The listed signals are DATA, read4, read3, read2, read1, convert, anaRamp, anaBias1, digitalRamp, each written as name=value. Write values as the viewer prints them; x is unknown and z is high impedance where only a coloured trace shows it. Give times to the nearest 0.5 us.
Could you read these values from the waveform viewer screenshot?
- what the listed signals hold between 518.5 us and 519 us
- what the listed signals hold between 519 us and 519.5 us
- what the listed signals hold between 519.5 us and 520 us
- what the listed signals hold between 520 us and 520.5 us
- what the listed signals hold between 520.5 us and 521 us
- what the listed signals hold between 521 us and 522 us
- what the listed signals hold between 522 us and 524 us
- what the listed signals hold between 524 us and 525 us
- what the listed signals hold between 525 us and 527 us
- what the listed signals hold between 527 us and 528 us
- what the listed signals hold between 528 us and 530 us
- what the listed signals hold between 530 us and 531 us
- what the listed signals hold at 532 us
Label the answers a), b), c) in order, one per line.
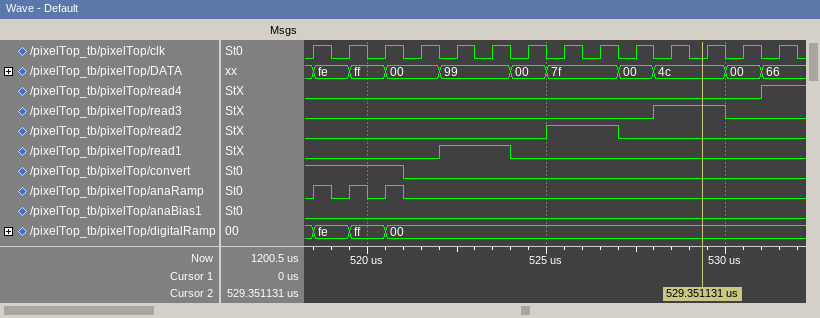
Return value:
a) DATA=fe, read4=0, read3=0, read2=0, read1=0, convert=1, anaRamp=1, anaBias1=0, digitalRamp=fe
b) DATA=fe, read4=0, read3=0, read2=0, read1=0, convert=1, anaRamp=0, anaBias1=0, digitalRamp=fe
c) DATA=ff, read4=0, read3=0, read2=0, read1=0, convert=1, anaRamp=1, anaBias1=0, digitalRamp=ff
d) DATA=ff, read4=0, read3=0, read2=0, read1=0, convert=1, anaRamp=0, anaBias1=0, digitalRamp=ff
e) DATA=00, read4=0, read3=0, read2=0, read1=0, convert=1, anaRamp=1, anaBias1=0, digitalRamp=00
f) DATA=00, read4=0, read3=0, read2=0, read1=0, convert=0, anaRamp=0, anaBias1=0, digitalRamp=00
g) DATA=99, read4=0, read3=0, read2=0, read1=1, convert=0, anaRamp=0, anaBias1=0, digitalRamp=00
h) DATA=00, read4=0, read3=0, read2=0, read1=0, convert=0, anaRamp=0, anaBias1=0, digitalRamp=00
i) DATA=7f, read4=0, read3=0, read2=1, read1=0, convert=0, anaRamp=0, anaBias1=0, digitalRamp=00
j) DATA=00, read4=0, read3=0, read2=0, read1=0, convert=0, anaRamp=0, anaBias1=0, digitalRamp=00
k) DATA=4c, read4=0, read3=1, read2=0, read1=0, convert=0, anaRamp=0, anaBias1=0, digitalRamp=00
l) DATA=00, read4=0, read3=0, read2=0, read1=0, convert=0, anaRamp=0, anaBias1=0, digitalRamp=00
m) DATA=66, read4=1, read3=0, read2=0, read1=0, convert=0, anaRamp=0, anaBias1=0, digitalRamp=00
